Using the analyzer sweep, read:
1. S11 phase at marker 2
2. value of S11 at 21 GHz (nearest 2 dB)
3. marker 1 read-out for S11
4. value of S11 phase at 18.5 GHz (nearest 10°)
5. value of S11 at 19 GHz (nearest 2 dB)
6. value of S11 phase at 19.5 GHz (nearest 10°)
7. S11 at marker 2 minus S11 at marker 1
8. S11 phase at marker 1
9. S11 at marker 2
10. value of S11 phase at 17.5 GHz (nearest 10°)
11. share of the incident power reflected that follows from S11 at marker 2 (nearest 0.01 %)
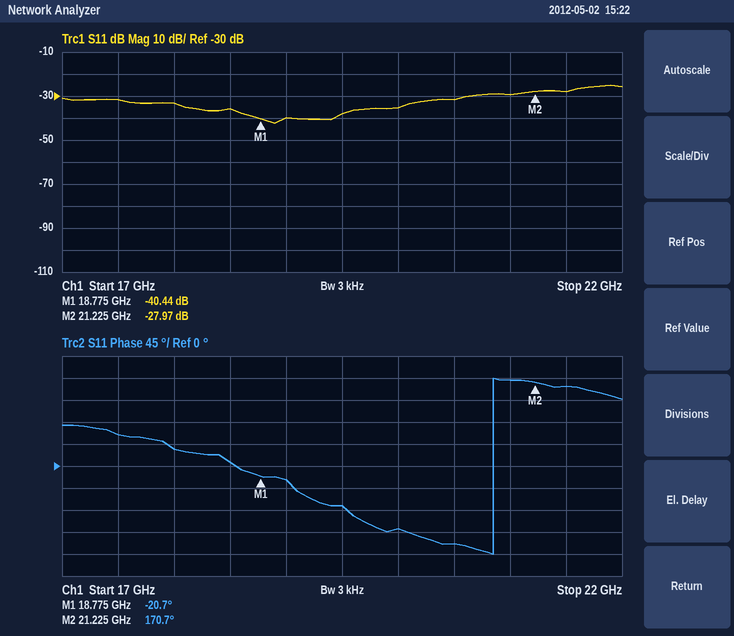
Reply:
170.7°
-30 dB
-40.44 dB
10°
-40 dB
-80°
12.47 dB
-20.7°
-27.97 dB
60°
0.16 %
